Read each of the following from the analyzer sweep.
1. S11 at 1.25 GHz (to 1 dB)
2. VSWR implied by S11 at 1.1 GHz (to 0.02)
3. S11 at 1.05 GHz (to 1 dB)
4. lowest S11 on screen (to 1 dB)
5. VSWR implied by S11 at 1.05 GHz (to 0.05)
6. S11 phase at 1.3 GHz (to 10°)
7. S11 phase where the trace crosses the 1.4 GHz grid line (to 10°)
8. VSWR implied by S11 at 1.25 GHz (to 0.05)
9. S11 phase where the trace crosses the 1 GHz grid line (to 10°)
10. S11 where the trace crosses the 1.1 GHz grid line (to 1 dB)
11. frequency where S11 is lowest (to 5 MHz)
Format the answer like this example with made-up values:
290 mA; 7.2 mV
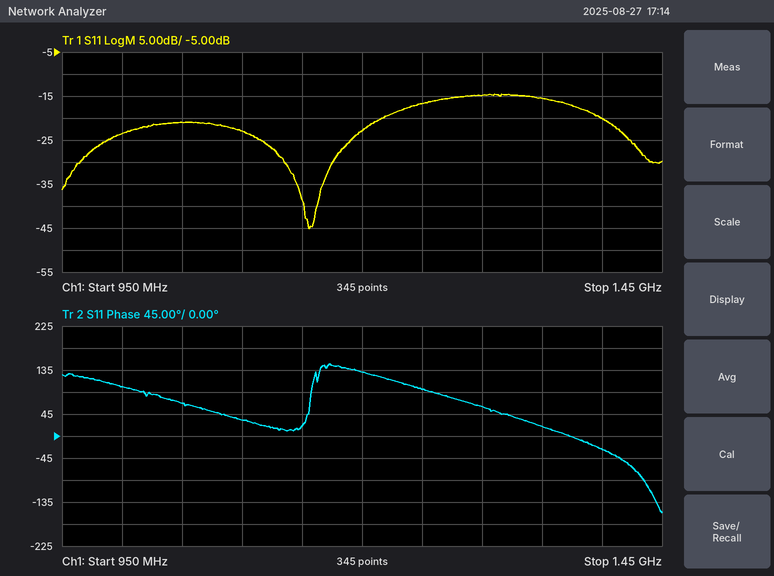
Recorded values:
-17 dB; 1.16; -21 dB; -45 dB; 1.20; 60°; -30°; 1.35; 100°; -23 dB; 1.155 GHz
